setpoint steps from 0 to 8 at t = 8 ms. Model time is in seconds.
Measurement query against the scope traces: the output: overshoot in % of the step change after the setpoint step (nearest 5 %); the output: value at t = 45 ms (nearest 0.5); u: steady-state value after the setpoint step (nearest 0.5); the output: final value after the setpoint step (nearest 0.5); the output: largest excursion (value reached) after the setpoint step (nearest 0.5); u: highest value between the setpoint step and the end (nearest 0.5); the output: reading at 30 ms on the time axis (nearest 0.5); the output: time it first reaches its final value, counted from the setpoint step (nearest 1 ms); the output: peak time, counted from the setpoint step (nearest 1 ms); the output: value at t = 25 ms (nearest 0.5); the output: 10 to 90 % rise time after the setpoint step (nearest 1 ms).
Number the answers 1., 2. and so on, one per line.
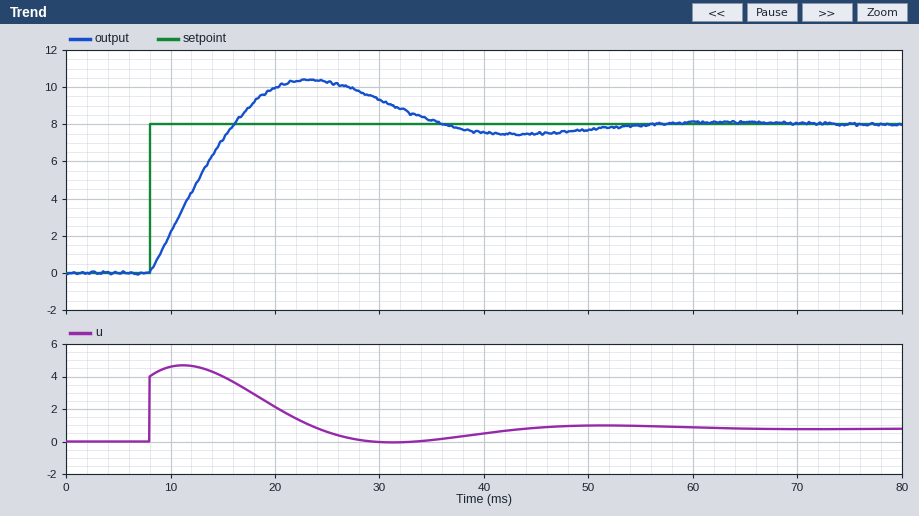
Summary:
1. 30 %
2. 7.5
3. 1.0
4. 8.0
5. 10.5
6. 4.5
7. 9.5
8. 8 ms
9. 15 ms
10. 10.5
11. 6 ms
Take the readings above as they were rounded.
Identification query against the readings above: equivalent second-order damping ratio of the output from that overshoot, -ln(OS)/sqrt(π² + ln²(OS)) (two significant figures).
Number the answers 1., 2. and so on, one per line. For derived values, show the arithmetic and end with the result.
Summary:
1. ln(0.3) = -1.204; 1.204 / sqrt(9.870 + 1.450) = 0.36
